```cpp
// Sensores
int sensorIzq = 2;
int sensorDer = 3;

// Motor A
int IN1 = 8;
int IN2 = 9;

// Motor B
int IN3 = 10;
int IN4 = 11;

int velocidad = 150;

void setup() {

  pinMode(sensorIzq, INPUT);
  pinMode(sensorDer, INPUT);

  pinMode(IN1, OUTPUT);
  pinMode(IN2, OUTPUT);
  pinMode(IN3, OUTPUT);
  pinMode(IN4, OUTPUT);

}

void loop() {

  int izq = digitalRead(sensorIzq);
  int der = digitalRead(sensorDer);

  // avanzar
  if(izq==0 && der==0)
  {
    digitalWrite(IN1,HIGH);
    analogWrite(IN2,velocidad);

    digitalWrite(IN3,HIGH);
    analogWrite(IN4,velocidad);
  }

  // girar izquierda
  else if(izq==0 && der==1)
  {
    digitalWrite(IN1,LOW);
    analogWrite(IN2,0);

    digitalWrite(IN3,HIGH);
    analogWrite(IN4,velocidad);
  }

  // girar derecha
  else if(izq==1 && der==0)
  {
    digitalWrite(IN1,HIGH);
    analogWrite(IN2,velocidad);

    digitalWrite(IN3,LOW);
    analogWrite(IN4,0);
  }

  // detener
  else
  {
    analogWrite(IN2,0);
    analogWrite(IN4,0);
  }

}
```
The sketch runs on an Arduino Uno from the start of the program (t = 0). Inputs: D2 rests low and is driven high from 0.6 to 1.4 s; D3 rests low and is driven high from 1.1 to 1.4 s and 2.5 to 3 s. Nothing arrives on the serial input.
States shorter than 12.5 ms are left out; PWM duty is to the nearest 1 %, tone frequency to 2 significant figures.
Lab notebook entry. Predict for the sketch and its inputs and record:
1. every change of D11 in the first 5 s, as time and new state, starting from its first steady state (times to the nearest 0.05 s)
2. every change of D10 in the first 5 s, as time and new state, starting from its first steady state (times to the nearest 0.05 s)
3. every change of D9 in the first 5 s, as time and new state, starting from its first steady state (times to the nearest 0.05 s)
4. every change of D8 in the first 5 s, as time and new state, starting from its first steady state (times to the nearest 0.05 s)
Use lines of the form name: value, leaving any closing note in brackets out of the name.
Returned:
every change of D11 in the first 5 s, as time and new state, starting from its first steady state: 0 s PWM 59 %; 0.6 s low; 1.4 s PWM 59 %
every change of D10 in the first 5 s, as time and new state, starting from its first steady state: 0 s high; 0.6 s low; 1.4 s high
every change of D9 in the first 5 s, as time and new state, starting from its first steady state: 0 s PWM 59 %; 1.1 s low; 1.4 s PWM 59 %; 2.5 s low; 3 s PWM 59 %
every change of D8 in the first 5 s, as time and new state, starting from its first steady state: 0 s high; 2.5 s low; 3 s high
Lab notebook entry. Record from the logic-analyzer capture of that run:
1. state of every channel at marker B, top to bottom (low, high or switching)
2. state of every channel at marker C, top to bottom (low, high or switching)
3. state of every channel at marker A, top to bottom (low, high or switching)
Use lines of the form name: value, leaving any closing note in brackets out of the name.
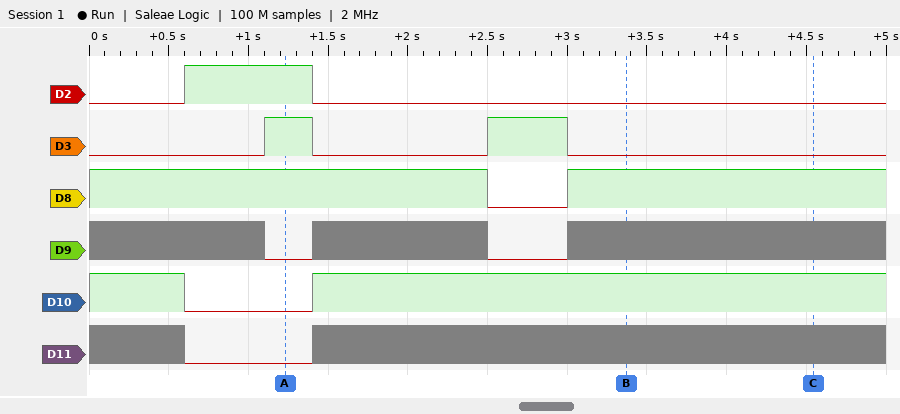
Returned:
state of every channel at marker B, top to bottom: D2 low, D3 low, D8 high, D9 switching, D10 high, D11 switching
state of every channel at marker C, top to bottom: D2 low, D3 low, D8 high, D9 switching, D10 high, D11 switching
state of every channel at marker A, top to bottom: D2 high, D3 high, D8 high, D9 low, D10 low, D11 low
